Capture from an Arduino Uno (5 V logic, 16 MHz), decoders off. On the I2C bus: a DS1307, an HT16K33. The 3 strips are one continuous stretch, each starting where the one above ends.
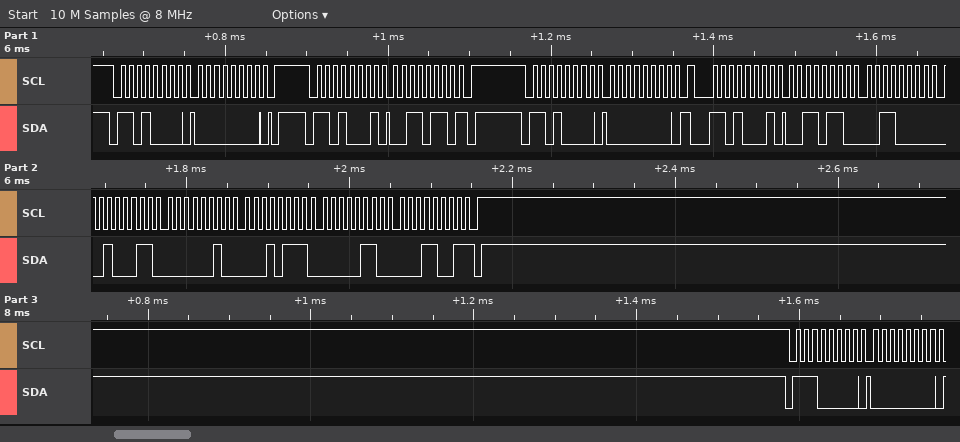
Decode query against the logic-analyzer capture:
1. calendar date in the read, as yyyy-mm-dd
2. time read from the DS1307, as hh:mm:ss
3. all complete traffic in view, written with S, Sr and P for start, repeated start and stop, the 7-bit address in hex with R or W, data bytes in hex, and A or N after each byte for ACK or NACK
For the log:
2019-06-17
23:30:36
S 68W A 00 A P S 68R A 36 N P S 68W A 00 A Sr 68R A 36 A 30 A 23 A 02 A 17 A 06 A 19 N P S 70W A 00 A
